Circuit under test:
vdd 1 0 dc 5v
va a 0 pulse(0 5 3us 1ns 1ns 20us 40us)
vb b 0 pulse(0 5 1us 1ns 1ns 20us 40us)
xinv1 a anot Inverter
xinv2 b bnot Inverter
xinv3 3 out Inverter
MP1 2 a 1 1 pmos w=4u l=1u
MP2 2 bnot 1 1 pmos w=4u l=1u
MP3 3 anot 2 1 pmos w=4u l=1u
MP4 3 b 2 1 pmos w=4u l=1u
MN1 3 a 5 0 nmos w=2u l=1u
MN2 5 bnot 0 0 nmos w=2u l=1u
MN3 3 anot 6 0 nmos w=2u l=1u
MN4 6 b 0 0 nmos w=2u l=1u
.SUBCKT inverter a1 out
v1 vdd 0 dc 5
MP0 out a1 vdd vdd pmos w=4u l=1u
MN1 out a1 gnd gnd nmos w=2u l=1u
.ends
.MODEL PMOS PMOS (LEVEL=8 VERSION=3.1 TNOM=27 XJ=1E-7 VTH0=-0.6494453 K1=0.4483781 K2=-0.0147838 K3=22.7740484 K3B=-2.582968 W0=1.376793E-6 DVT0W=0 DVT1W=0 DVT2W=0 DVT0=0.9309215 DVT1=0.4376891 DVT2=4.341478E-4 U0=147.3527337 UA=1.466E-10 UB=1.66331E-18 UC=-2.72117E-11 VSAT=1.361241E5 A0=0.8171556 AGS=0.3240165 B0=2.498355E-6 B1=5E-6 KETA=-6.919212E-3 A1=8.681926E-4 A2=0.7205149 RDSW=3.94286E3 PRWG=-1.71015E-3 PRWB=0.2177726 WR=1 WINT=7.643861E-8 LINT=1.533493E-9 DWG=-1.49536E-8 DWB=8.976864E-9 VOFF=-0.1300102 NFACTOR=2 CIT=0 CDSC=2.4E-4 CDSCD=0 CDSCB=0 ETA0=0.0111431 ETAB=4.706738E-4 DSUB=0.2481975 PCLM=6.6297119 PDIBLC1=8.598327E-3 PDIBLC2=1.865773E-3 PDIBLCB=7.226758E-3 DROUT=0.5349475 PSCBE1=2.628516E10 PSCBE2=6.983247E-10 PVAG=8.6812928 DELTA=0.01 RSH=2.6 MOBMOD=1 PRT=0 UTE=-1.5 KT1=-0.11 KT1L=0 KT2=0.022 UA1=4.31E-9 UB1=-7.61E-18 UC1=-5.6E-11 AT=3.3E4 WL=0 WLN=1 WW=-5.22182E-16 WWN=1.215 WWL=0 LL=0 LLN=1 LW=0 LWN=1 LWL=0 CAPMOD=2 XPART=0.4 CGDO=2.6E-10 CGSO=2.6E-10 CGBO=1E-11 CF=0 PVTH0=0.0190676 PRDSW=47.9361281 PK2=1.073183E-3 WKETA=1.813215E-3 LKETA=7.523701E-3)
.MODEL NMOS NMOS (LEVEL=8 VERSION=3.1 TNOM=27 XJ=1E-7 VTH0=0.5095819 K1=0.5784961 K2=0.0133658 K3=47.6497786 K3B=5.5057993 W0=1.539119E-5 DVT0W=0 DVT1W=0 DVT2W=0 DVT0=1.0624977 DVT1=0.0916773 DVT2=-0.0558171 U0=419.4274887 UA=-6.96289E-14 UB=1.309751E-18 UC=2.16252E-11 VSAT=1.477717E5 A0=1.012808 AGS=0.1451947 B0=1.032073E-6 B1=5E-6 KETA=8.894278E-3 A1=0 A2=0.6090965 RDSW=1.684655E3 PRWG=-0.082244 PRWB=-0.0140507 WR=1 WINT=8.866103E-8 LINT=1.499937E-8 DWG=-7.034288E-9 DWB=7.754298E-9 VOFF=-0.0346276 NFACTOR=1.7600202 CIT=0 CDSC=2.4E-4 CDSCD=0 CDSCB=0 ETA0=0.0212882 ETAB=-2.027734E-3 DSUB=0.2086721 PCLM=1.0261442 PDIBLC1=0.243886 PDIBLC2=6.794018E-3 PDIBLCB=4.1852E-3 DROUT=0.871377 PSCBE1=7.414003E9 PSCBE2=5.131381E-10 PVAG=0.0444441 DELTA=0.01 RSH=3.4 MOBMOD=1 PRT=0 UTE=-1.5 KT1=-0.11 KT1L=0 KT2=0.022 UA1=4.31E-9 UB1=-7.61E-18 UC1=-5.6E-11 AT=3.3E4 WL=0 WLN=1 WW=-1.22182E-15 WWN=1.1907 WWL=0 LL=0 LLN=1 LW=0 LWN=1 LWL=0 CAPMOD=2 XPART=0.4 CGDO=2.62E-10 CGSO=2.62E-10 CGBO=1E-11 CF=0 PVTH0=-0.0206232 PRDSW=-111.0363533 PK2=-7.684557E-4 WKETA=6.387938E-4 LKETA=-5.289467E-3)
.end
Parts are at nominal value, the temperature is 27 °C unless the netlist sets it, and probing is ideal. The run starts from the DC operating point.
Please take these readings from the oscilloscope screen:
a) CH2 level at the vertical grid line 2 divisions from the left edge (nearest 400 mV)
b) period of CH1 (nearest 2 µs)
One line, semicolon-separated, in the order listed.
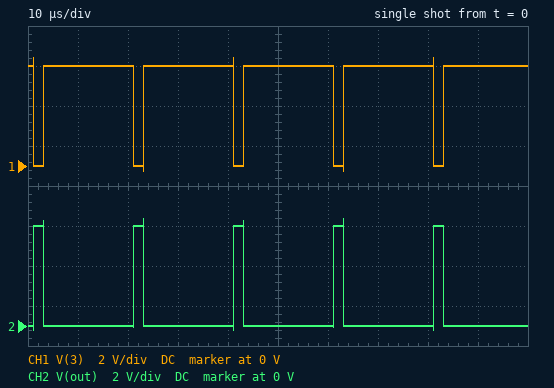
0 V; 20 µs
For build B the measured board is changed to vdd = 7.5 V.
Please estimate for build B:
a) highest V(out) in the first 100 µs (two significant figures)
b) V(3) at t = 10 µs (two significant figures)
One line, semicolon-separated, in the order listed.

4.4 V; 7.5 V
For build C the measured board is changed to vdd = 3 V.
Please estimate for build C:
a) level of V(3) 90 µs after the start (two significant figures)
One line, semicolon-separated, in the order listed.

3.0 V
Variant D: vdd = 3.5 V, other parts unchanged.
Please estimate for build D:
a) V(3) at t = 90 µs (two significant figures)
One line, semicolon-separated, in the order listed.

3.5 V
